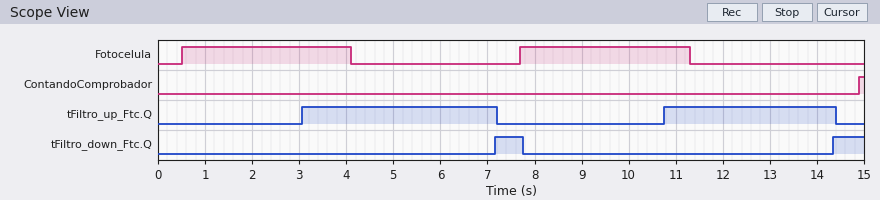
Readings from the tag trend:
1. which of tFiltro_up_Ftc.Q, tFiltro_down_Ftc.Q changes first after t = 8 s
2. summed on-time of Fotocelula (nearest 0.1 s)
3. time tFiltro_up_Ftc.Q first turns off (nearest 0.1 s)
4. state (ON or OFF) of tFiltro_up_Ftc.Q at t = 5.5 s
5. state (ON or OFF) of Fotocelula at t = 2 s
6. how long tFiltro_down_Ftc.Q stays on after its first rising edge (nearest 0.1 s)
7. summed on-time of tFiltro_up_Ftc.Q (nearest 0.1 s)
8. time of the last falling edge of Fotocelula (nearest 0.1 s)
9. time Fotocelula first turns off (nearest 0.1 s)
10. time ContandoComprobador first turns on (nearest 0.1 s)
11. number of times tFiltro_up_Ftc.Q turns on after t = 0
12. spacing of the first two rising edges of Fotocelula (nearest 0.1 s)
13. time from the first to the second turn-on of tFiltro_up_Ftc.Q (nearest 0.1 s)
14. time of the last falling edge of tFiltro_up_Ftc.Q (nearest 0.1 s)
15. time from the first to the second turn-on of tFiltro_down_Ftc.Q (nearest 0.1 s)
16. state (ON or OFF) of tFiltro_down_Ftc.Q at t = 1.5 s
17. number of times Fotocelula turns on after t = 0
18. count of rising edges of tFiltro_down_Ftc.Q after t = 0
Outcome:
tFiltro_up_Ftc.Q
7.2 s
7.2 s
ON
ON
0.6 s
7.8 s
11.3 s
4.1 s
14.9 s
2
7.2 s
7.7 s
14.4 s
7.2 s
OFF
2
2
